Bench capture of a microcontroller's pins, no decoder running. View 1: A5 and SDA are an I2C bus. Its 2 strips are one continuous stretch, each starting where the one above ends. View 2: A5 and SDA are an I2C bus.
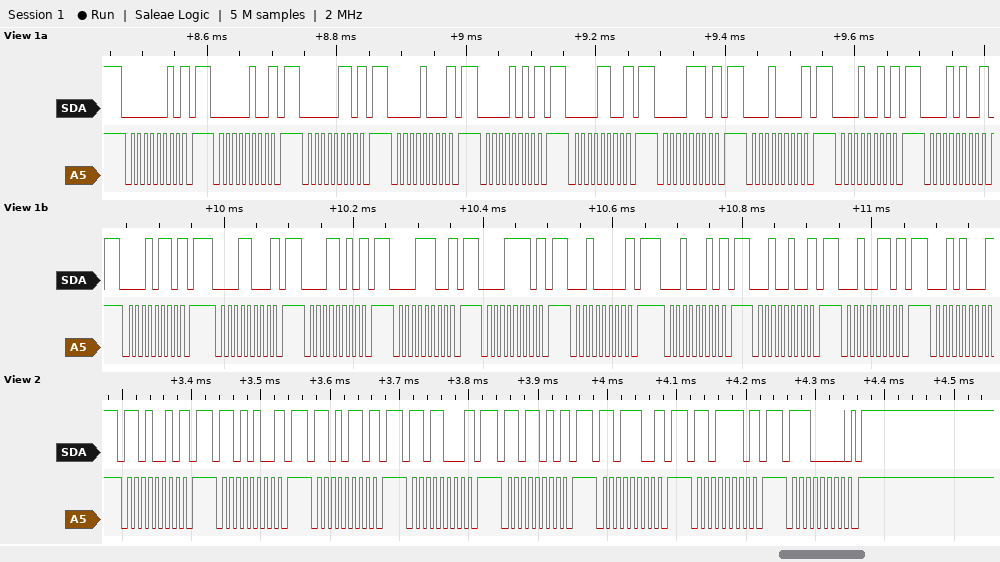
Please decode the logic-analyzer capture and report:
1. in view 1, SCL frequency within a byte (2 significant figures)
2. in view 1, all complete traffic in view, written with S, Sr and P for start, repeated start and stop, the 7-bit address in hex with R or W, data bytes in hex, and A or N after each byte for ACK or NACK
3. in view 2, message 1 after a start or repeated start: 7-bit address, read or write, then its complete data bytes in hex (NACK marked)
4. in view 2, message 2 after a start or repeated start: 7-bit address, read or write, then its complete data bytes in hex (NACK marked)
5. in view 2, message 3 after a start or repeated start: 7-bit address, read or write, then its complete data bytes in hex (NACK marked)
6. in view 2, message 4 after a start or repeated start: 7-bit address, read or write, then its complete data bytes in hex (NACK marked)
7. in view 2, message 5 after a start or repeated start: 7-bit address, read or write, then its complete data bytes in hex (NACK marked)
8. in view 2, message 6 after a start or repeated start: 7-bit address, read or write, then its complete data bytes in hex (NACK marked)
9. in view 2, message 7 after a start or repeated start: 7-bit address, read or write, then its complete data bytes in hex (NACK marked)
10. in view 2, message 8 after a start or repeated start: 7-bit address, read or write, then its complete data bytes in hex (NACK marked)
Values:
100 kHz
S 01W N P S 02W N P S 03W N P S 04W N P S 05W N P S 06W N P S 07W N P S 08W N P S 09W N P S 0AW N P S 0BW N P S 0CW N P S 0DW N P S 0EW N P S 0FW N P S 10W N P S 11W N P S 12W N P S 13W N P S 14W N
0x69 write NACK
0x6A write NACK
0x6B write NACK
0x6C write NACK
0x6D write NACK
0x6E write NACK
0x6F write NACK
0x70 write
